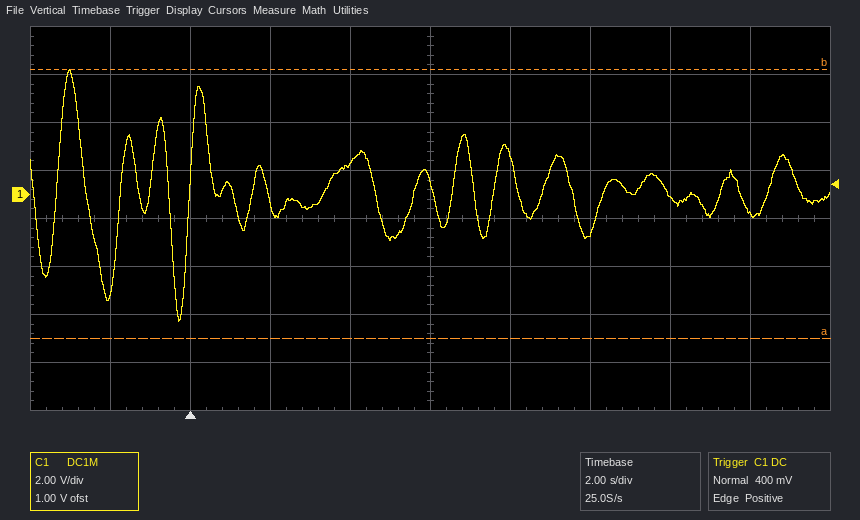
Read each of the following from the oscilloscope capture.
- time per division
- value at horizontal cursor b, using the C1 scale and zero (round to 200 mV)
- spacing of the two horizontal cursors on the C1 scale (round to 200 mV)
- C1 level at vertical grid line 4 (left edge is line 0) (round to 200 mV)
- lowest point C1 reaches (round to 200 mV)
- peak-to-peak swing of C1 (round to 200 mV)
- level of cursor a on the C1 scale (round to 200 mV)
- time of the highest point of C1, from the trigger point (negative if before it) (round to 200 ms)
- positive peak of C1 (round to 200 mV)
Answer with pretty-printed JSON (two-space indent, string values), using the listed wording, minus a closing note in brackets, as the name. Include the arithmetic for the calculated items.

{
  "time per division": "2 s",
  "value at horizontal cursor b, using the C1 scale and zero": "5.2 V",
  "spacing of the two horizontal cursors on the C1 scale": "11.2 V",
  "C1 level at vertical grid line 4 (left edge is line 0)": "1.4 V",
  "lowest point C1 reaches": "-5.2 V",
  "peak-to-peak swing of C1": "5.2 V − (-5.2 V) = 10.4 V",
  "level of cursor a on the C1 scale": "-6.0 V",
  "time of the highest point of C1, from the trigger point (negative if before it)": "-3.0 s",
  "positive peak of C1": "5.2 V"
}
